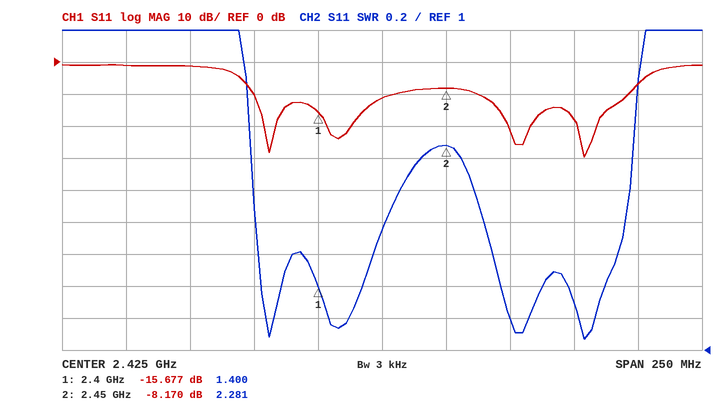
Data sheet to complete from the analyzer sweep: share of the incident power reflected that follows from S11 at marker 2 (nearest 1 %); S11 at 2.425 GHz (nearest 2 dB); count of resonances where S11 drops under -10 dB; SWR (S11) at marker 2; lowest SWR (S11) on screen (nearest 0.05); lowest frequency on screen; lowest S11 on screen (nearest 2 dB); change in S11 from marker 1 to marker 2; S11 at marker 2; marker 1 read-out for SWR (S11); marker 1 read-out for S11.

15 %
-12 dB
4
2.281
1.05
2.3 GHz
-30 dB
7.507 dB
-8.170 dB
1.400
-15.677 dB
